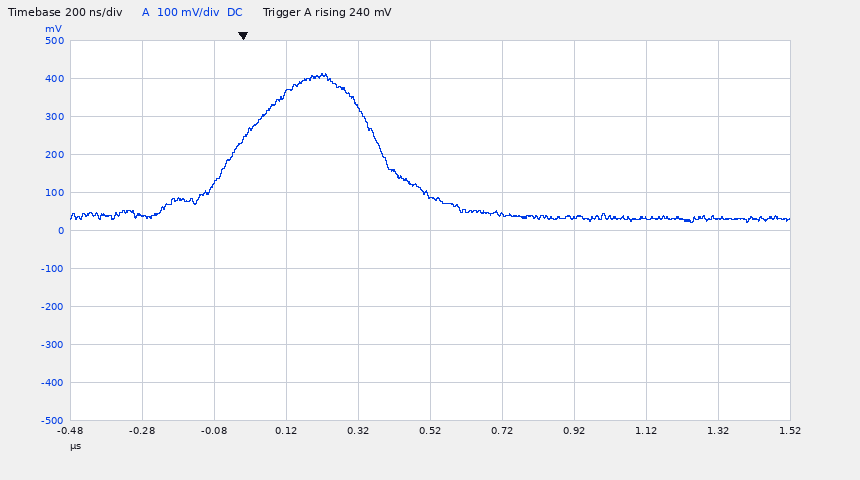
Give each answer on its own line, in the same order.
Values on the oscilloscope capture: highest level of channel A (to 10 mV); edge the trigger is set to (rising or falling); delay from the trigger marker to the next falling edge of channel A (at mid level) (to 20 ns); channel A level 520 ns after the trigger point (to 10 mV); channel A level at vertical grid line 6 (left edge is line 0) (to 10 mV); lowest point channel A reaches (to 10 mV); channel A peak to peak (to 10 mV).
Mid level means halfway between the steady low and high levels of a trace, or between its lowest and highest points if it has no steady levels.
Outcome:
410 mV
rising
380 ns
90 mV
40 mV
20 mV
390 mV
